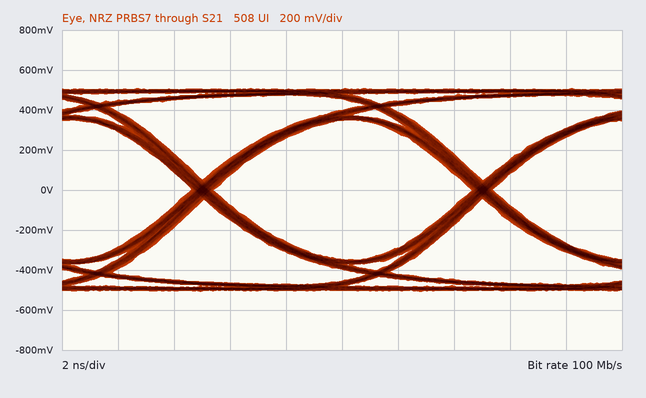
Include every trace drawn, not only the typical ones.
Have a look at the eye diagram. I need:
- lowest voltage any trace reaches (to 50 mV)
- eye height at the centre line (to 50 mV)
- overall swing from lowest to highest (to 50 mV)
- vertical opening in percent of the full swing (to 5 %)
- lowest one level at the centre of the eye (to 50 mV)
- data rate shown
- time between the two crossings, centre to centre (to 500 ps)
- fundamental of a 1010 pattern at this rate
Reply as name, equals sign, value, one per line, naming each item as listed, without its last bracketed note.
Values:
lowest voltage any trace reaches = -500 mV
eye height at the centre line = 700 mV
overall swing from lowest to highest = 1.00 V
vertical opening in percent of the full swing = 70 %
lowest one level at the centre of the eye = 350 mV
data rate shown = 100 Mb/s
time between the two crossings, centre to centre = 10.0 ns
fundamental of a 1010 pattern at this rate = 50 MHz
